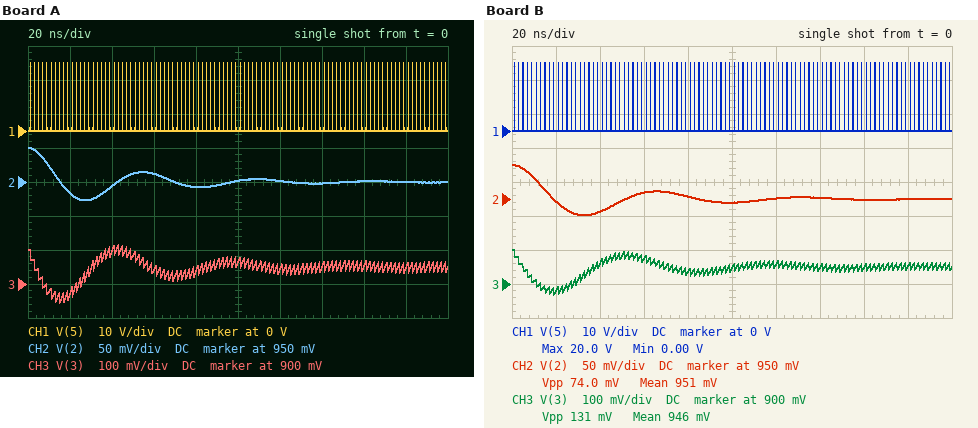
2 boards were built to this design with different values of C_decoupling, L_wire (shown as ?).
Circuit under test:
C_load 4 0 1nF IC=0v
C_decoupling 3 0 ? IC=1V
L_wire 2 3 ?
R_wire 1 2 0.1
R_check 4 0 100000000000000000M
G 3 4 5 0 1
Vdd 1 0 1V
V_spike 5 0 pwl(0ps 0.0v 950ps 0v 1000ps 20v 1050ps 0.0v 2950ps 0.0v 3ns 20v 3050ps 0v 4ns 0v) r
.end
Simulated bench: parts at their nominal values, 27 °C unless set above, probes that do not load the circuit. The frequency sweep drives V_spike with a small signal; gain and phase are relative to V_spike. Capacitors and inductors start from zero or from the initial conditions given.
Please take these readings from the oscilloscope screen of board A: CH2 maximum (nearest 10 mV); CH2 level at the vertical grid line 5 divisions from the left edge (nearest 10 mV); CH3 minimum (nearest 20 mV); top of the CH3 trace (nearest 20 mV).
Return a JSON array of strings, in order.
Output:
["1.00 V", "950 mV", "840 mV", "1.02 V"]
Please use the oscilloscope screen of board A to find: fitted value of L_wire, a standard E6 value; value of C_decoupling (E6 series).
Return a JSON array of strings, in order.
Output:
["2.2 nH", "33 nF"]
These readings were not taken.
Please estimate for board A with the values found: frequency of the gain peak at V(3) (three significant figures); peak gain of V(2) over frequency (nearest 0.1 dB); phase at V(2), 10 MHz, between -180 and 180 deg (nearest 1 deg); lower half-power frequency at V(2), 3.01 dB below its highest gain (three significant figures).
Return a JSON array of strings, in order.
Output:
["18.6 MHz", "-11.6 dB", "164 deg", "13.8 MHz"]
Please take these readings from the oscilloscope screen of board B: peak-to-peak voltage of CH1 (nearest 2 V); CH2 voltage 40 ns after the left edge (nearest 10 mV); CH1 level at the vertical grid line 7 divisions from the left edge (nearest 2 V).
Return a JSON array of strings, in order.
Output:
["20 V", "930 mV", "0 V"]
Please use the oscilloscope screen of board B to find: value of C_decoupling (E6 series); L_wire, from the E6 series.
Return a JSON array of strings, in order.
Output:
["47 nF", "2.2 nH"]
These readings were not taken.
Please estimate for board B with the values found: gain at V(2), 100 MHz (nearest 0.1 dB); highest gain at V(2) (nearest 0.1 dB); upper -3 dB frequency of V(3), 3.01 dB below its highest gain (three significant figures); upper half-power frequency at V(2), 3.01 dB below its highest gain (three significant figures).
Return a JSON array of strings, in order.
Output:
["-52.0 dB", "-13.1 dB", "19.4 MHz", "18.1 MHz"]
